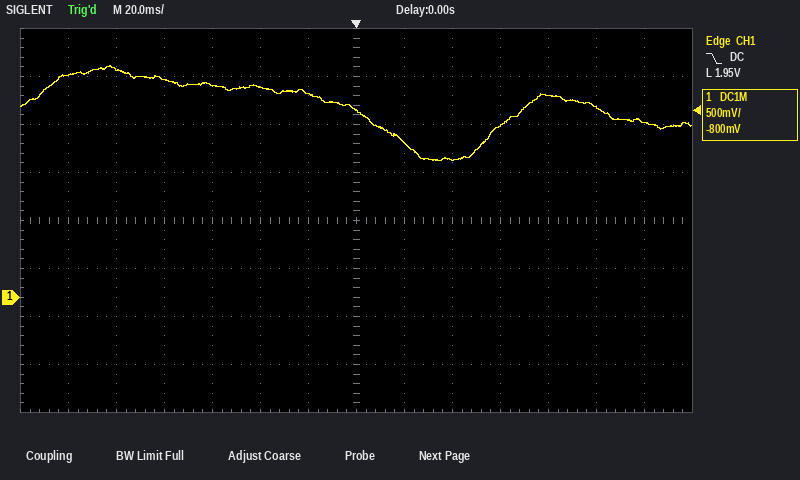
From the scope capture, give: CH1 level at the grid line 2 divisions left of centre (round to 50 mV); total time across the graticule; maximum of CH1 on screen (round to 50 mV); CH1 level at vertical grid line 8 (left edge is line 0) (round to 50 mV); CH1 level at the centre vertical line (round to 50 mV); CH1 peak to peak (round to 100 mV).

2.20 V
280 ms
2.40 V
1.60 V
1.95 V
1.00 V
